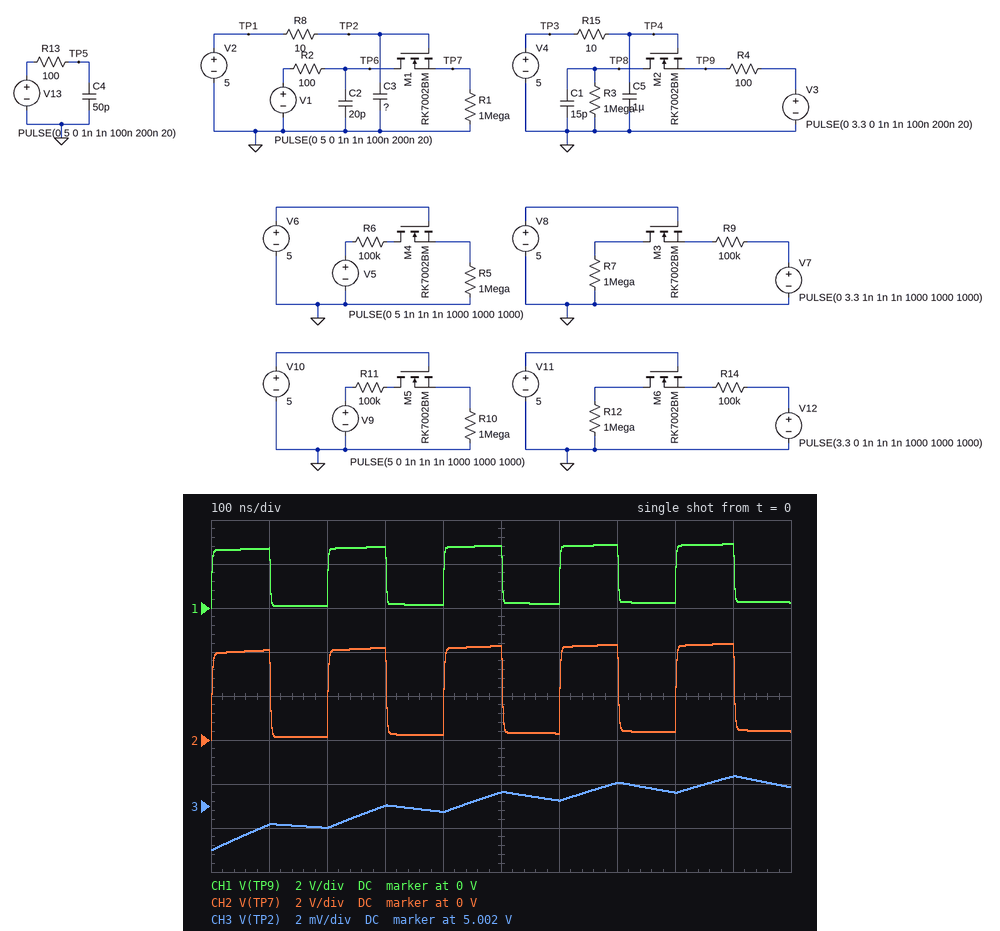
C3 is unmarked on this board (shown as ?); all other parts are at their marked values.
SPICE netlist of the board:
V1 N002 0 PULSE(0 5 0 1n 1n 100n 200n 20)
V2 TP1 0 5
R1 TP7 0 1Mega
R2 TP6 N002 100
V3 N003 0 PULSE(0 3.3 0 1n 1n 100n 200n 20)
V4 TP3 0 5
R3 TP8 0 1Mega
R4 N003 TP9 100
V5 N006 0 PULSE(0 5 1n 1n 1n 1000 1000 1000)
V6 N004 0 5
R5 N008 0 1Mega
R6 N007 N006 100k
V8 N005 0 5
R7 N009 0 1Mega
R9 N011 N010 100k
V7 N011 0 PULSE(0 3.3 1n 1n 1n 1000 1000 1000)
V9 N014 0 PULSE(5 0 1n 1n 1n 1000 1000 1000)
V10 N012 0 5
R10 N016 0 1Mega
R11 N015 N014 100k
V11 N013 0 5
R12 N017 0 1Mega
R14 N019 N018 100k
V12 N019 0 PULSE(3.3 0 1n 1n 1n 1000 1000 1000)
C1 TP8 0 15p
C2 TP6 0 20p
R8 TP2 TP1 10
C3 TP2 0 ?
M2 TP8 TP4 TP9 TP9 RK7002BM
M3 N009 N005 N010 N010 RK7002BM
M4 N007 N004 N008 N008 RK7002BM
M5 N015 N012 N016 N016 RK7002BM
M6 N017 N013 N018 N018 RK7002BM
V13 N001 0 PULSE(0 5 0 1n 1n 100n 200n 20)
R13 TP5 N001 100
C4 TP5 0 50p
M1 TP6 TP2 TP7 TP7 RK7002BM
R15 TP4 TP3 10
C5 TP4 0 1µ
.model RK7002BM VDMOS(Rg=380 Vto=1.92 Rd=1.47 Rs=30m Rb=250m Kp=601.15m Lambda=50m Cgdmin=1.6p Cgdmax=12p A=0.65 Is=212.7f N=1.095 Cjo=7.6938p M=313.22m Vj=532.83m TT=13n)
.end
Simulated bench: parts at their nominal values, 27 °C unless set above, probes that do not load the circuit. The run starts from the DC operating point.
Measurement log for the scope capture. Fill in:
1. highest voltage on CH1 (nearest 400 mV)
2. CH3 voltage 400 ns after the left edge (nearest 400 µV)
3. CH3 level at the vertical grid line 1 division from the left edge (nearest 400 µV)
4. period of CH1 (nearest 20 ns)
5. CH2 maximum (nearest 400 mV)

2.8 V
5.0016 V
5.0012 V
200 ns
4.4 V
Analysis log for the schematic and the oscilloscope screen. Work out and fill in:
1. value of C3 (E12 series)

820 nF
